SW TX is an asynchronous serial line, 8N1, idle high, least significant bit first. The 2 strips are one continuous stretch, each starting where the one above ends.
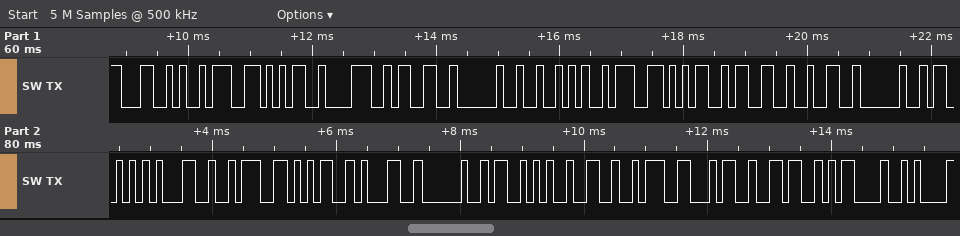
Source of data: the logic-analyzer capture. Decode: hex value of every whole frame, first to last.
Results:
4C 3A 35 38 33 20 52 3A 35 33 32 20 53 31 3A 35 31 20 53 32 3A 34 36 0D 0A
